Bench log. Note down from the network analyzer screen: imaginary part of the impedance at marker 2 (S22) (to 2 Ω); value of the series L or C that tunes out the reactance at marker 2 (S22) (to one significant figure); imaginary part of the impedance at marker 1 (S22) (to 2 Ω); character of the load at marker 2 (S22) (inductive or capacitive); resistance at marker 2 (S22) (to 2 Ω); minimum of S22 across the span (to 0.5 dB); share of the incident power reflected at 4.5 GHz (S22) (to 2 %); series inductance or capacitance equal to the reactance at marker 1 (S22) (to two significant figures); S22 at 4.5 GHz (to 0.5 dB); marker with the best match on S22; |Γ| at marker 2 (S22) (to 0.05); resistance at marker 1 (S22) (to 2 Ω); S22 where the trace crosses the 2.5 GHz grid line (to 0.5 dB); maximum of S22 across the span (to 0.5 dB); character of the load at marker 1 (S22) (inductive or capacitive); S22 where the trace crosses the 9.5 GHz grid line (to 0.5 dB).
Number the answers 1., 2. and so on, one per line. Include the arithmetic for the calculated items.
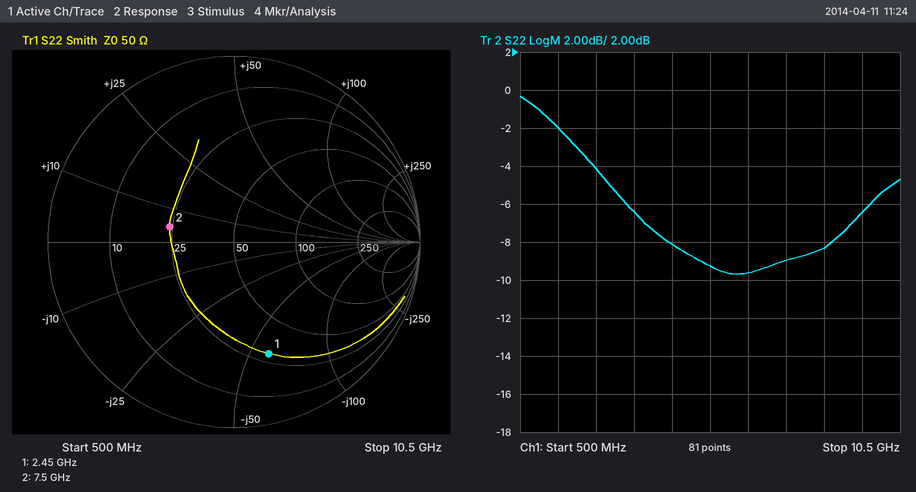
1. +4 Ω
2. C = 1/(2π × 7.5 GHz × 4 Ω) ≈ 5 pF
3. -58 Ω
4. inductive
5. 24 Ω
6. -9.5 dB
7. 10^(-8/10) ≈ 16 %
8. C = 1/(2π × 2.45 GHz × 58 Ω) ≈ 1.1 pF
9. -8.0 dB
10. marker 2
11. 0.35
12. 30 Ω
13. -4.0 dB
14. -0.5 dB
15. capacitive
16. -6.5 dB
